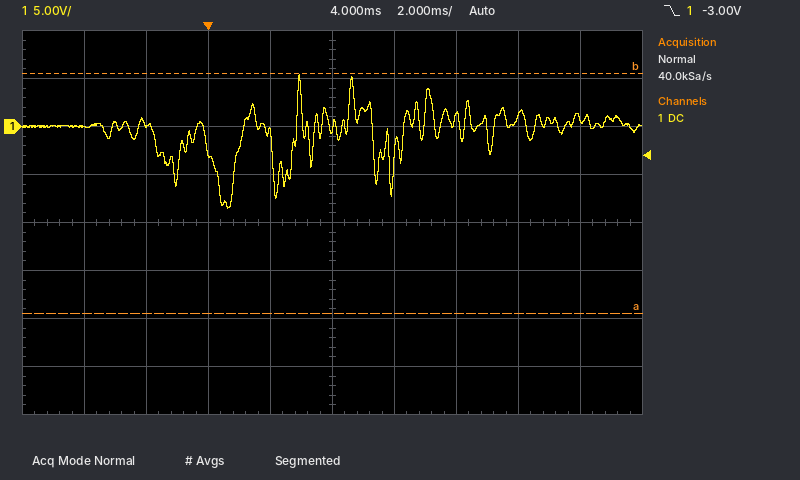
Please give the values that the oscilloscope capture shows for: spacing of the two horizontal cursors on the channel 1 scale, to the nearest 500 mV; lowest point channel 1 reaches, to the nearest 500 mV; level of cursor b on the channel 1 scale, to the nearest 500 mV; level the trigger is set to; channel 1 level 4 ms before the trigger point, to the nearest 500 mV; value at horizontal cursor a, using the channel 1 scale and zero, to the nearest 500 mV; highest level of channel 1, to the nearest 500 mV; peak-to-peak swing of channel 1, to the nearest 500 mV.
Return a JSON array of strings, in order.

["25.0 V", "-8.5 V", "5.5 V", "-3.00 V", "0.0 V", "-19.5 V", "5.5 V", "14.0 V"]
